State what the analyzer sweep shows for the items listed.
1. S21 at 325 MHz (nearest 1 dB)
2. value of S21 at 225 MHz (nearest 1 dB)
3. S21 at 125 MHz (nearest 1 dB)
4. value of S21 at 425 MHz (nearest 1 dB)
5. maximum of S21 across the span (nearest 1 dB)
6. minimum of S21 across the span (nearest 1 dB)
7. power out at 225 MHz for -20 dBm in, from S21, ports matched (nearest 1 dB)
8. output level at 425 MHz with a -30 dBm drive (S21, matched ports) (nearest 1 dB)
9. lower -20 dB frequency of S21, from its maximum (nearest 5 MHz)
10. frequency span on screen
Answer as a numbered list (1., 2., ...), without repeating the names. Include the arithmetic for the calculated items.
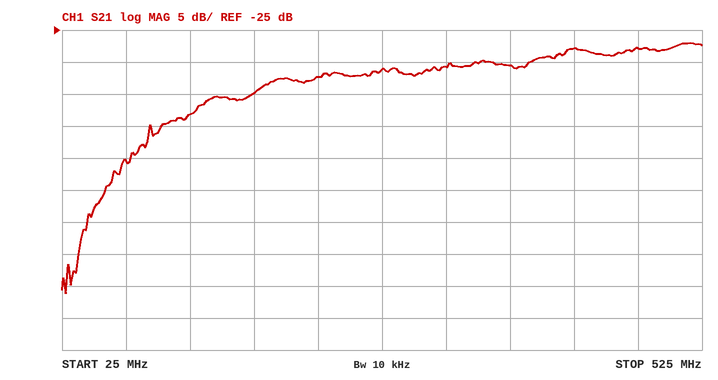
1. -31 dB
2. -32 dB
3. -38 dB
4. -28 dB
5. -27 dB
6. -66 dB
7. -20 dBm + (-32 dB) = -52 dBm
8. -30 dBm + (-28 dB) = -58 dBm
9. 70 MHz
10. 500 MHz
